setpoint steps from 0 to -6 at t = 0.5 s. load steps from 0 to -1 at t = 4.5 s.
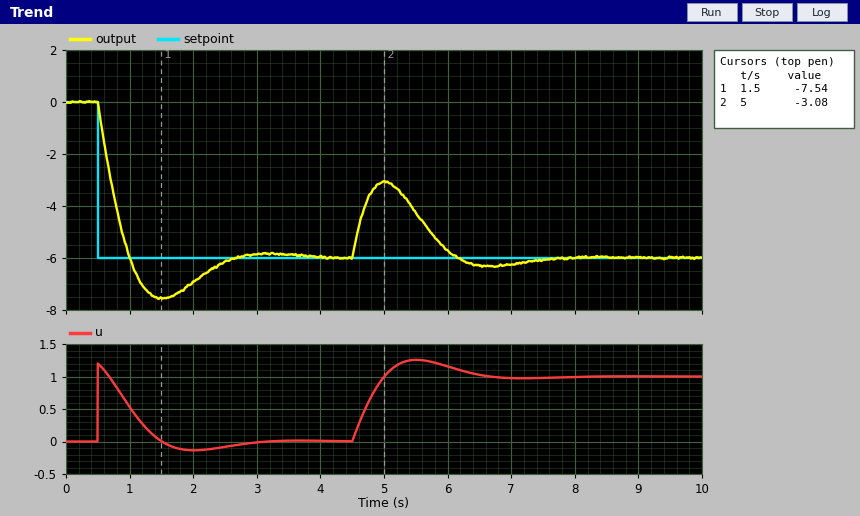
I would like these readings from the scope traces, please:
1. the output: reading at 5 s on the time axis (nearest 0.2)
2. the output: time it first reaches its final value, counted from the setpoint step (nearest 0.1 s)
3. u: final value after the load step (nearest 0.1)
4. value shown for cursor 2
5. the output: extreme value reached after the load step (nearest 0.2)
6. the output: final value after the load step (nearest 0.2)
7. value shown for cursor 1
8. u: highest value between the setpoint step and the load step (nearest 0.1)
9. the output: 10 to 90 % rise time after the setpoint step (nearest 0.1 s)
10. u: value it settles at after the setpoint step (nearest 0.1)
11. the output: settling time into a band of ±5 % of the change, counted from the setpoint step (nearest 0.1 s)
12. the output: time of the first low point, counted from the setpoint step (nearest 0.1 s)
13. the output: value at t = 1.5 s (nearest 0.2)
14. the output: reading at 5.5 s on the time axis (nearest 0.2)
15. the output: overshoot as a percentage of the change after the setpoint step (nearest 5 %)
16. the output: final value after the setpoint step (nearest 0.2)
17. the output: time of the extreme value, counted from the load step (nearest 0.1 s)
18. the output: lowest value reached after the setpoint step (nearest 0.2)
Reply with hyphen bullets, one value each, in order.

- -3.0
- 0.5 s
- 1.0
- -3.08
- -3.0
- -6.0
- -7.54
- 1.2
- 0.4 s
- 0.0
- 1.9 s
- 1.0 s
- -7.6
- -4.2
- 25 %
- -6.0
- 0.5 s
- -7.6
